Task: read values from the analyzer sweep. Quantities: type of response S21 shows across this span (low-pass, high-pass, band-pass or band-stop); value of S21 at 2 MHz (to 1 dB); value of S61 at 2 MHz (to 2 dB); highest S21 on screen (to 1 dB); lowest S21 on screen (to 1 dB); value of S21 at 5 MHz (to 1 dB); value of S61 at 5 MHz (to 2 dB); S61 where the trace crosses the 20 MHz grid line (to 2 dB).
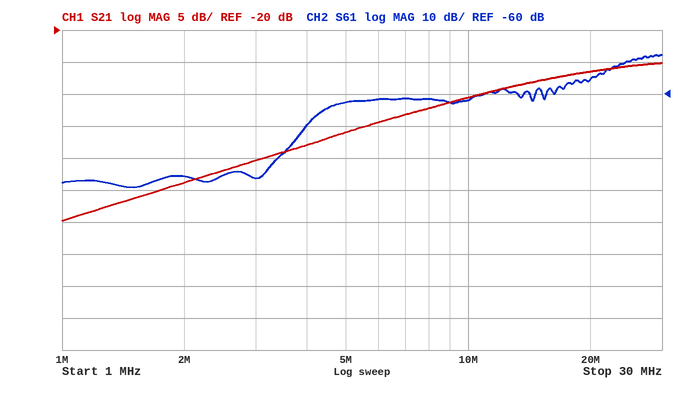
high-pass
-44 dB
-86 dB
-25 dB
-50 dB
-36 dB
-62 dB
-56 dB
